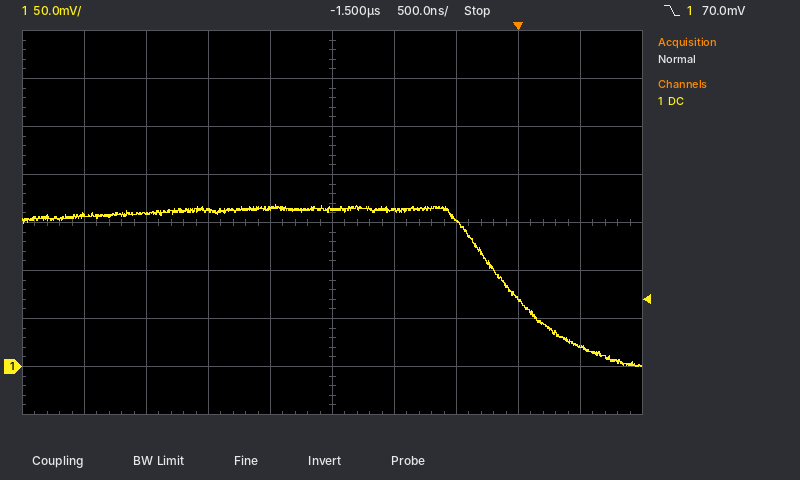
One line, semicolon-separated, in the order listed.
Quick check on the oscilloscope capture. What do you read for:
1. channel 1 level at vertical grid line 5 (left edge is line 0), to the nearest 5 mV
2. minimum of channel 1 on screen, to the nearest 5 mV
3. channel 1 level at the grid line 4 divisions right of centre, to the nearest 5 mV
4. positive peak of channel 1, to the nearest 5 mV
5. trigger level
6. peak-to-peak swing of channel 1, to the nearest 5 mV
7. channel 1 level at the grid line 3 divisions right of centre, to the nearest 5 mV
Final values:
165 mV; 0 mV; 20 mV; 170 mV; 70.0 mV; 170 mV; 70 mV
